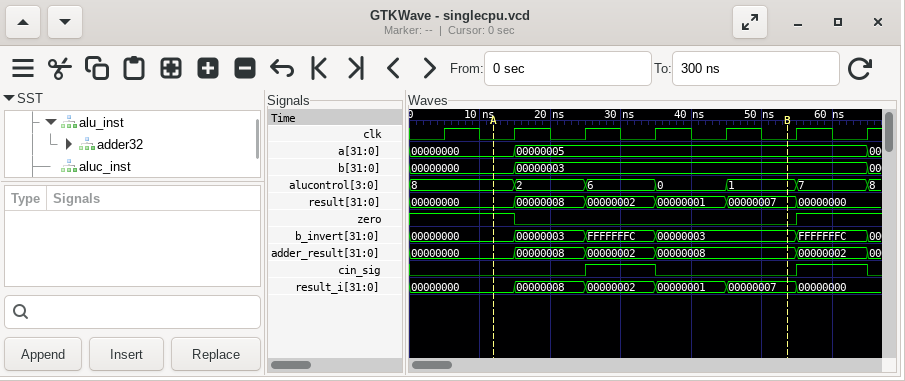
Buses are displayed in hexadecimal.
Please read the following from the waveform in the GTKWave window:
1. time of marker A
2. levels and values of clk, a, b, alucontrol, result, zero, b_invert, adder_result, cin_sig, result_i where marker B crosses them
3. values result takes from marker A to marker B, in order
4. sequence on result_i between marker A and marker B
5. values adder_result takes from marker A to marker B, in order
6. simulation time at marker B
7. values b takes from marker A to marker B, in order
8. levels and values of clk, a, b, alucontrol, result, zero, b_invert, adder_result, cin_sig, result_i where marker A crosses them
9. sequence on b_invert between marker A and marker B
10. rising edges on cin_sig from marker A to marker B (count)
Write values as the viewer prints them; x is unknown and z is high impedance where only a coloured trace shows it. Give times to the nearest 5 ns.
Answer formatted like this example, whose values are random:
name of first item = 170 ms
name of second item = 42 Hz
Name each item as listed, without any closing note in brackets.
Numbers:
time of marker A = 10 ns
levels and values of clk, a, b, alucontrol, result, zero, b_invert, adder_result, cin_sig, result_i where marker B crosses them = clk=0, a=00000005, b=00000003, alucontrol=1, result=00000007, zero=0, b_invert=00000003, adder_result=00000008, cin_sig=0, result_i=00000007
values result takes from marker A to marker B, in order = 00000000, 00000008, 00000002, 00000001, 00000007
sequence on result_i between marker A and marker B = 00000000, 00000008, 00000002, 00000001, 00000007
values adder_result takes from marker A to marker B, in order = 00000000, 00000008, 00000002, 00000008
simulation time at marker B = 55 ns
values b takes from marker A to marker B, in order = 00000000, 00000003
levels and values of clk, a, b, alucontrol, result, zero, b_invert, adder_result, cin_sig, result_i where marker A crosses them = clk=0, a=00000000, b=00000000, alucontrol=8, result=00000000, zero=1, b_invert=00000000, adder_result=00000000, cin_sig=0, result_i=00000000
sequence on b_invert between marker A and marker B = 00000000, 00000003, FFFFFFFC, 00000003
rising edges on cin_sig from marker A to marker B = 1
